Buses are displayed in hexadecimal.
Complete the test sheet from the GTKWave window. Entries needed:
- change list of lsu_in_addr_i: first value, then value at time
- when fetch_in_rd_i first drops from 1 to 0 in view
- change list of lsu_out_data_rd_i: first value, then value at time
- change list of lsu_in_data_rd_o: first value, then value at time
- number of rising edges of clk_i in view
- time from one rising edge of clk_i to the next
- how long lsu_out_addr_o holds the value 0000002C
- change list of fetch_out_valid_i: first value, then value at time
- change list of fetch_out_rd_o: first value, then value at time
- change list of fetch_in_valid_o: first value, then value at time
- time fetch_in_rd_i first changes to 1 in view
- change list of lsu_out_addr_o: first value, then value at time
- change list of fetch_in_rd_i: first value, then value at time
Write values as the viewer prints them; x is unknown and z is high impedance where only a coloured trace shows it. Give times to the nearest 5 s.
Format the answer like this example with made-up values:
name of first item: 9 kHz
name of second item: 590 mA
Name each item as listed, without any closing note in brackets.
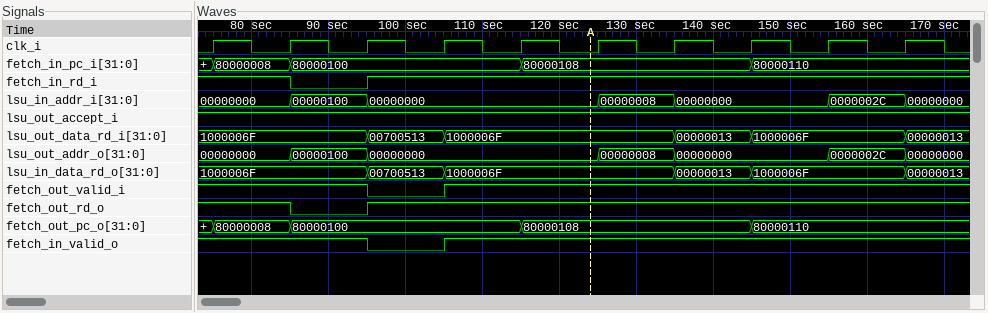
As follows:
change list of lsu_in_addr_i: first value, then value at time: 00000000, 00000100 at 85 s, 00000000 at 95 s, 00000008 at 125 s, 00000000 at 135 s, 0000002C at 155 s, 00000000 at 165 s
when fetch_in_rd_i first drops from 1 to 0 in view: 85 s
change list of lsu_out_data_rd_i: first value, then value at time: 1000006F, 00700513 at 95 s, 1000006F at 105 s, 00000013 at 135 s, 1000006F at 145 s, 00000013 at 165 s
change list of lsu_in_data_rd_o: first value, then value at time: 1000006F, 00700513 at 95 s, 1000006F at 105 s, 00000013 at 135 s, 1000006F at 145 s, 00000013 at 165 s
number of rising edges of clk_i in view: 10
time from one rising edge of clk_i to the next: 10 s
how long lsu_out_addr_o holds the value 0000002C: 10 s
change list of fetch_out_valid_i: first value, then value at time: 1, 0 at 95 s, 1 at 105 s
change list of fetch_out_rd_o: first value, then value at time: 1, 0 at 85 s, 1 at 95 s
change list of fetch_in_valid_o: first value, then value at time: 1, 0 at 95 s, 1 at 105 s
time fetch_in_rd_i first changes to 1 in view: 95 s
change list of lsu_out_addr_o: first value, then value at time: 00000000, 00000100 at 85 s, 00000000 at 95 s, 00000008 at 125 s, 00000000 at 135 s, 0000002C at 155 s, 00000000 at 165 s
change list of fetch_in_rd_i: first value, then value at time: 1, 0 at 85 s, 1 at 95 s
